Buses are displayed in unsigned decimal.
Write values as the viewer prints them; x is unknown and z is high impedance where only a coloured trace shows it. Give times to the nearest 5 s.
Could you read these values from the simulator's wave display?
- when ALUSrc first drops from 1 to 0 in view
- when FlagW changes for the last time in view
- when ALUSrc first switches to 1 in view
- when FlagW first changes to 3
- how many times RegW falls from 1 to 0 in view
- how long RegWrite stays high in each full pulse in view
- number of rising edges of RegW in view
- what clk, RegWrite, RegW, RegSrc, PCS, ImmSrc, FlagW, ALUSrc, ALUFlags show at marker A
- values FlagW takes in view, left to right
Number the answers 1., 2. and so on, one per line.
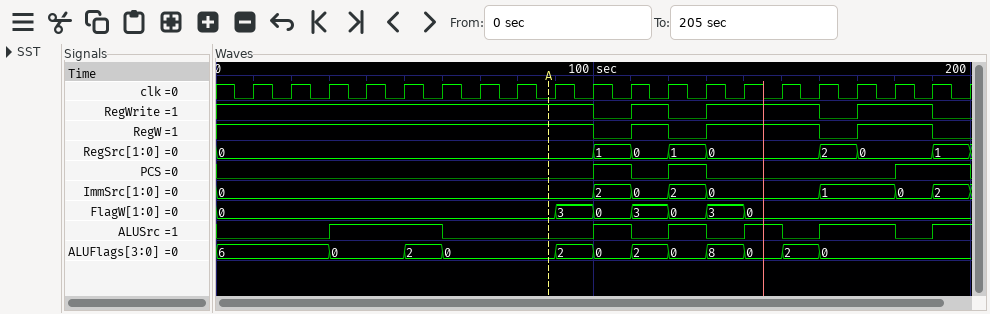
1. 60 s
2. 140 s
3. 30 s
4. 90 s
5. 4
6. 10 s, 30 s, 20 s
7. 3
8. clk=0, RegWrite=1, RegW=1, RegSrc=0, PCS=0, ImmSrc=0, FlagW=0, ALUSrc=0, ALUFlags=0
9. 0, 3, 0, 3, 0, 3, 0
